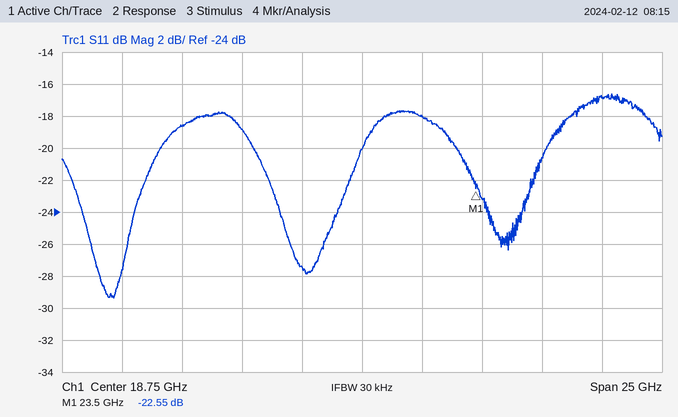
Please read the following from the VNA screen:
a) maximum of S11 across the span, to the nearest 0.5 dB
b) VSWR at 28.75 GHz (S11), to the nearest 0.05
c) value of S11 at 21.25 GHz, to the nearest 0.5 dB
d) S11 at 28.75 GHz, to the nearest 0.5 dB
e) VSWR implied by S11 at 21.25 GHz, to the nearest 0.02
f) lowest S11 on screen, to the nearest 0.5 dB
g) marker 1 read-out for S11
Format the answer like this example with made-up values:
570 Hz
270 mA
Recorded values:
-16.5 dB
1.35
-18.0 dB
-17.0 dB
1.28
-29.5 dB
-22.55 dB
